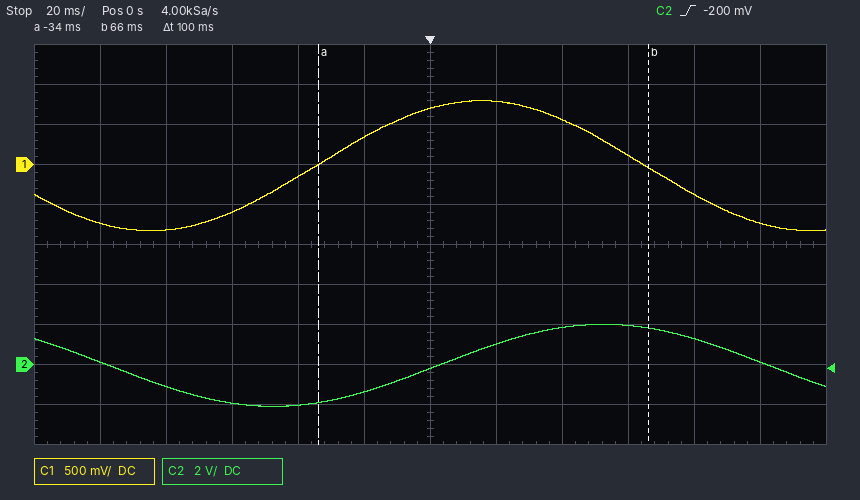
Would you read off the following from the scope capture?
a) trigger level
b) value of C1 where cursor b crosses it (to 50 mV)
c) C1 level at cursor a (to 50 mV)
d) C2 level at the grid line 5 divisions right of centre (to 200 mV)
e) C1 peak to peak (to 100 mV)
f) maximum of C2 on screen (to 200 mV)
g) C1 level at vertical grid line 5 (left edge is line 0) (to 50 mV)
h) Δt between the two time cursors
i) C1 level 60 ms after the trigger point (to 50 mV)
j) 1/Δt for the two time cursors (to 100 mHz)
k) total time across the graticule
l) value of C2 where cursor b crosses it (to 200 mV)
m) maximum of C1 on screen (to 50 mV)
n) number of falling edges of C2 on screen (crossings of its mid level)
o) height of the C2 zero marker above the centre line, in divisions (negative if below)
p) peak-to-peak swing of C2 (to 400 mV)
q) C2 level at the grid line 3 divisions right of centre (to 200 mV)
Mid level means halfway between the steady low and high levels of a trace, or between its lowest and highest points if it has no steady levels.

-200 mV
-50 mV
0 mV
200 mV
1.60 V
2.0 V
350 mV
100 ms
100 mV
10.0 Hz
240 ms
1.8 V
800 mV
2
-3.0 div
4.0 V
2.0 V
